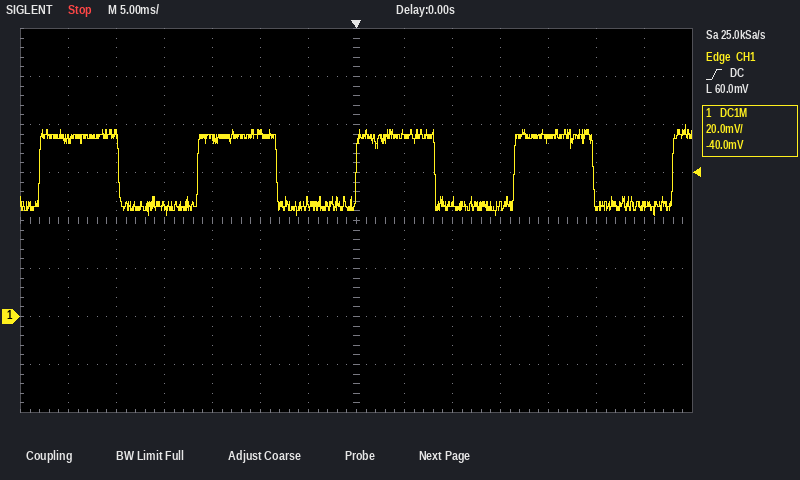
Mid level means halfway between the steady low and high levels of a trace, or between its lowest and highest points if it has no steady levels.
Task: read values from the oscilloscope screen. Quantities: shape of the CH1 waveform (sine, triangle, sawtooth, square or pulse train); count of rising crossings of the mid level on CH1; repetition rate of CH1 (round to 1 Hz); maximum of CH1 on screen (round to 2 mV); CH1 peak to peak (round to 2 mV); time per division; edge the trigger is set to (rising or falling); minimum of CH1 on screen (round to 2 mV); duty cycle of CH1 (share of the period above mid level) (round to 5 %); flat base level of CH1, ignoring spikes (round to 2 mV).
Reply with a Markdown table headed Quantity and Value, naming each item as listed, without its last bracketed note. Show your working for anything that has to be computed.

| Quantity | Value |
|---|---|
| shape of the CH1 waveform | square |
| count of rising crossings of the mid level on CH1 | 5 |
| repetition rate of CH1 | 61 Hz |
| maximum of CH1 on screen | 80 mV |
| CH1 peak to peak | 80 mV − (42 mV) = 38 mV |
| time per division | 5 ms |
| edge the trigger is set to | rising |
| minimum of CH1 on screen | 42 mV |
| duty cycle of CH1 (share of the period above mid level) | 50 % |
| flat base level of CH1, ignoring spikes | 46 mV |
